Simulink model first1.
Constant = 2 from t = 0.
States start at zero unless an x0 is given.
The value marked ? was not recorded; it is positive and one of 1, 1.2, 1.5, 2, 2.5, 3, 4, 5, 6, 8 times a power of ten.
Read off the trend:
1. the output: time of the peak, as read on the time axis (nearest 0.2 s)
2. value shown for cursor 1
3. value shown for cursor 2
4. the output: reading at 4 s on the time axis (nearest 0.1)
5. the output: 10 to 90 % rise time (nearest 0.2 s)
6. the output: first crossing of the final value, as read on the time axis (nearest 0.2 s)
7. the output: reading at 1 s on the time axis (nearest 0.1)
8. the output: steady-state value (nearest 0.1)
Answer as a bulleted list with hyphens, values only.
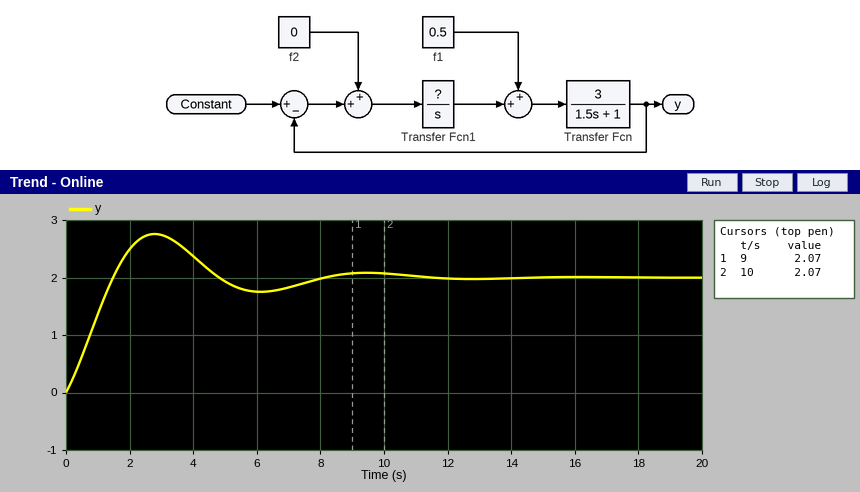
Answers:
- 2.8 s
- 2.07
- 2.07
- 2.4
- 1.2 s
- 1.4 s
- 1.4
- 2.0
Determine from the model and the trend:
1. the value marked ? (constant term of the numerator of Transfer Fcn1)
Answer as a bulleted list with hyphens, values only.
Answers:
- 0.5
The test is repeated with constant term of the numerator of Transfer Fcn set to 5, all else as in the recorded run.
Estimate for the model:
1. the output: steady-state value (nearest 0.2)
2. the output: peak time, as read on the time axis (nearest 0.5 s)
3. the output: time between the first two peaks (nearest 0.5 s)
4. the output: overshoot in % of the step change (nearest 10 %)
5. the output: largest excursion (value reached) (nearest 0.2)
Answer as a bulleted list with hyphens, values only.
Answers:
- 2.0
- 2.0 s
- 5.0 s
- 50 %
- 3.0
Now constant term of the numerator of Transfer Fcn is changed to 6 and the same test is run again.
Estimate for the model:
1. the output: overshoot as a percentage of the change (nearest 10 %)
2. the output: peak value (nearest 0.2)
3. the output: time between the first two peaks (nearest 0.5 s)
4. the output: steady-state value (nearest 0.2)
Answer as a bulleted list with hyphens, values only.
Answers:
- 60 %
- 3.2
- 4.5 s
- 2.0
